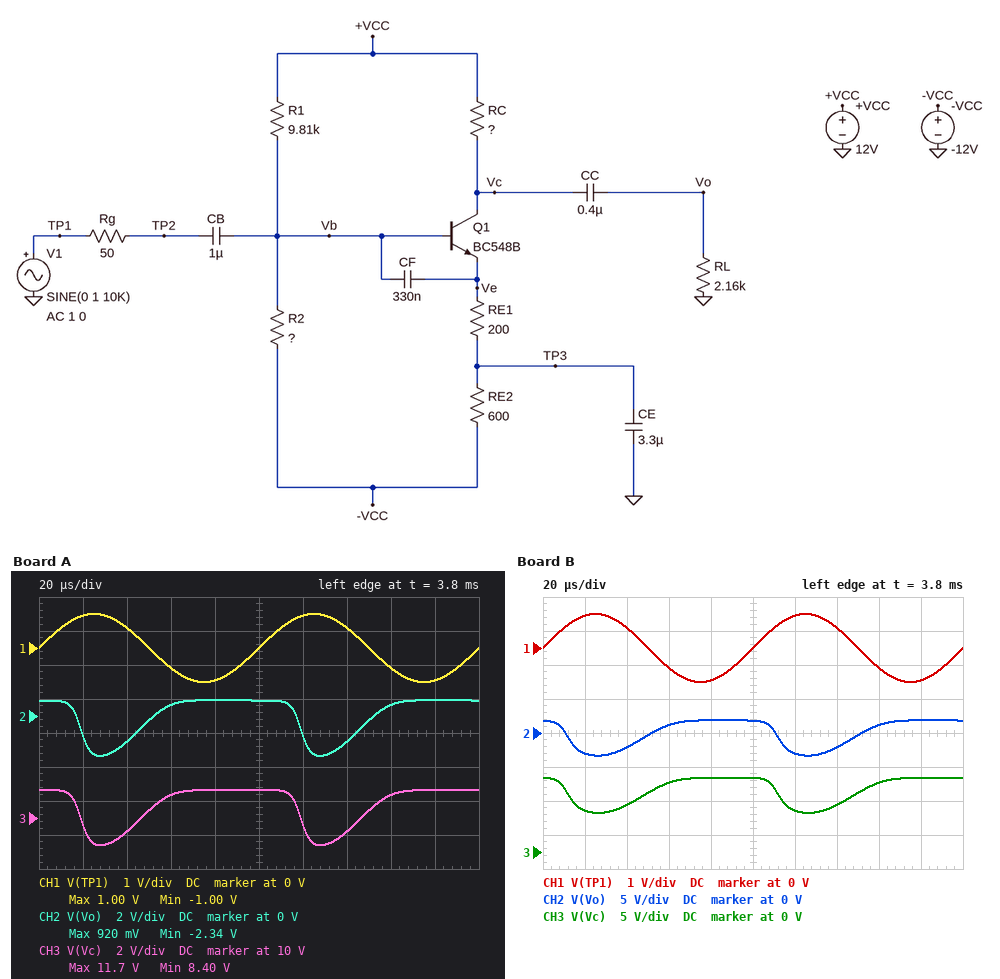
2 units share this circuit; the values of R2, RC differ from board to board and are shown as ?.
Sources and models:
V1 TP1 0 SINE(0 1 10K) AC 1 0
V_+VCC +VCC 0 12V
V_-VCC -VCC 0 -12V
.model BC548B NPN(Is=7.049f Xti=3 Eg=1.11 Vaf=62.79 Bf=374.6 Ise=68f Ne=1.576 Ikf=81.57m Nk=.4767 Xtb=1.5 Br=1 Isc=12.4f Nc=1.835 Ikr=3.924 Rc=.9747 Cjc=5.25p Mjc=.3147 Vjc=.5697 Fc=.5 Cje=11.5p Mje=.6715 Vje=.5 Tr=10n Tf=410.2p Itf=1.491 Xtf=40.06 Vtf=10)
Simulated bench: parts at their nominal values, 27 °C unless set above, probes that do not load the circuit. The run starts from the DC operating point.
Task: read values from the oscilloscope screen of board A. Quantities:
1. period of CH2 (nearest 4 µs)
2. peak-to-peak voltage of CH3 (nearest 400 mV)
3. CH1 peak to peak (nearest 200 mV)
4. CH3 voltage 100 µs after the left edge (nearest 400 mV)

100 µs
3.2 V
2.0 V
11.6 V
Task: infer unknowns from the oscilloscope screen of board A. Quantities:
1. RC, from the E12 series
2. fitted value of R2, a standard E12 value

820 Ω
820 Ω
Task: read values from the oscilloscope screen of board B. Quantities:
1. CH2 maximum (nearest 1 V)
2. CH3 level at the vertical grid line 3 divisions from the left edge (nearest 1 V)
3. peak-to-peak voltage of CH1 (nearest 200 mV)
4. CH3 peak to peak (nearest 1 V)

2 V
10 V
2.0 V
5 V
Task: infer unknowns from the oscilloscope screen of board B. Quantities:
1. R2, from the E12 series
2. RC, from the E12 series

1.2 kΩ
1.2 kΩ
